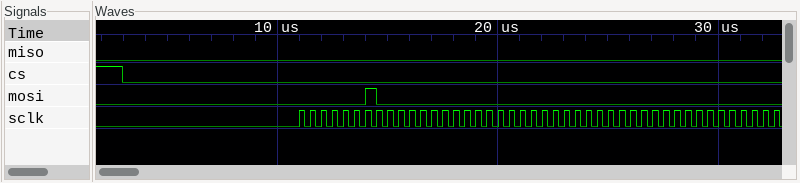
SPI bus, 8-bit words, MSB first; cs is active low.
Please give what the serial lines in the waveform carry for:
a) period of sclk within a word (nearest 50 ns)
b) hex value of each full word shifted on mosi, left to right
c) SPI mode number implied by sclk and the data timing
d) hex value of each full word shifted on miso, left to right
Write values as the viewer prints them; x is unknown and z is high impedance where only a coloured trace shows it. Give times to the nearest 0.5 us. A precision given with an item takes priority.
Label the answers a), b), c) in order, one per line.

a) 500 ns
b) 02, 00, 00, 00, 00
c) 1
d) 00, 00, 00, 00, 00
